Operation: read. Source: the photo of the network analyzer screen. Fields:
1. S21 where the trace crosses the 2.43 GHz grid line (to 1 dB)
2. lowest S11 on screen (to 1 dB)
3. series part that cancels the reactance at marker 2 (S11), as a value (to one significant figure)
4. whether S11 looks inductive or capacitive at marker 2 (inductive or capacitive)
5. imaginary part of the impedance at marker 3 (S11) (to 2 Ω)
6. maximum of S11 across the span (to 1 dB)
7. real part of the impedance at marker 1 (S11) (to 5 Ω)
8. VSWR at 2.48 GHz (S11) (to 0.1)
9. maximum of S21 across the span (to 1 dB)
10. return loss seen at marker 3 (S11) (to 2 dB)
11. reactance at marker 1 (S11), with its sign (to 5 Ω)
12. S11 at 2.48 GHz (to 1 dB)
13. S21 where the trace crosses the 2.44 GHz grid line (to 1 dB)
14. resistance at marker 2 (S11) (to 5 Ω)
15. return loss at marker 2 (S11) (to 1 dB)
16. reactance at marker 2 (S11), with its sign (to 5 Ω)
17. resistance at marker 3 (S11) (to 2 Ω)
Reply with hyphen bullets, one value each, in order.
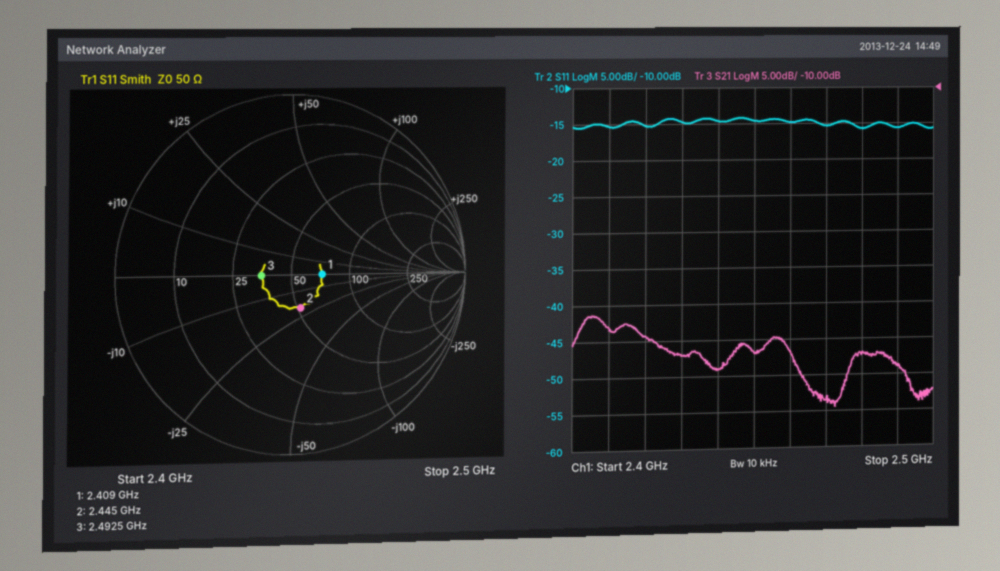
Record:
- -47 dB
- -16 dB
- 1 nH
- capacitive
- 0 Ω
- -14 dB
- 70 Ω
- 1.4
- -41 dB
- 16 dB
- 0 Ω
- -16 dB
- -49 dB
- 50 Ω
- 14 dB
- -20 Ω
- 36 Ω
